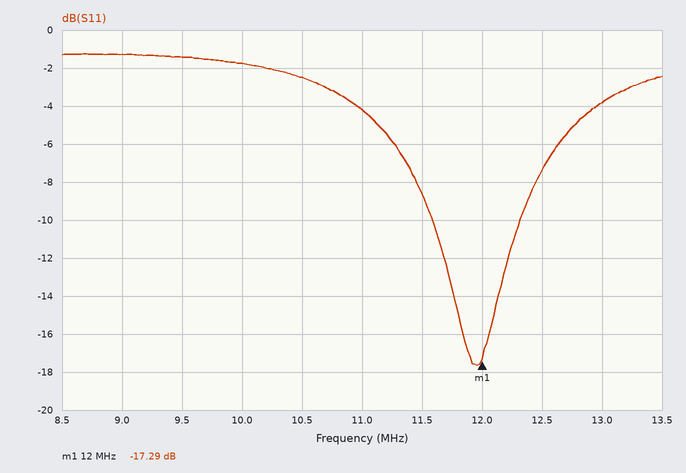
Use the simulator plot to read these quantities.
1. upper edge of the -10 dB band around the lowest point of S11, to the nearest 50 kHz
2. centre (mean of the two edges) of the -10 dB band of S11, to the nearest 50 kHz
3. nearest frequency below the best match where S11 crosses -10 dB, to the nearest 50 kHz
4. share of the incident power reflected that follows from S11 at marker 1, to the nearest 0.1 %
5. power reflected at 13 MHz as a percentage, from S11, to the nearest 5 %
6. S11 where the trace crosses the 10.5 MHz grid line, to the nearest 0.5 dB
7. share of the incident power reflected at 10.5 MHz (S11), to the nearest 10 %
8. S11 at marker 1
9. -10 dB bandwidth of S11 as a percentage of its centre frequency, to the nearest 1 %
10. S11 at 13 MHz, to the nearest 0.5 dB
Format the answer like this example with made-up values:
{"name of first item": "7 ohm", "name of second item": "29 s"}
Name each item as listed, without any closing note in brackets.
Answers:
{"upper edge of the -10 dB band around the lowest point of S11, to the nearest 50 kHz": "12.30 MHz", "centre (mean of the two edges) of the -10 dB band of S11, to the nearest 50 kHz": "11.95 MHz", "nearest frequency below the best match where S11 crosses -10 dB, to the nearest 50 kHz": "11.60 MHz", "share of the incident power reflected that follows from S11 at marker 1, to the nearest 0.1 %": "1.9 %", "power reflected at 13 MHz as a percentage, from S11, to the nearest 5 %": "40 %", "S11 where the trace crosses the 10.5 MHz grid line, to the nearest 0.5 dB": "-2.5 dB", "share of the incident power reflected at 10.5 MHz (S11), to the nearest 10 %": "60 %", "S11 at marker 1": "-17.29 dB", "-10 dB bandwidth of S11 as a percentage of its centre frequency, to the nearest 1 %": "6 %", "S11 at 13 MHz, to the nearest 0.5 dB": "-4.0 dB"}
